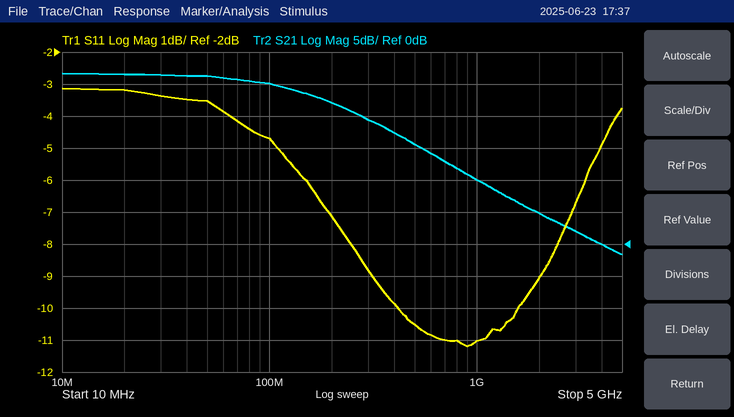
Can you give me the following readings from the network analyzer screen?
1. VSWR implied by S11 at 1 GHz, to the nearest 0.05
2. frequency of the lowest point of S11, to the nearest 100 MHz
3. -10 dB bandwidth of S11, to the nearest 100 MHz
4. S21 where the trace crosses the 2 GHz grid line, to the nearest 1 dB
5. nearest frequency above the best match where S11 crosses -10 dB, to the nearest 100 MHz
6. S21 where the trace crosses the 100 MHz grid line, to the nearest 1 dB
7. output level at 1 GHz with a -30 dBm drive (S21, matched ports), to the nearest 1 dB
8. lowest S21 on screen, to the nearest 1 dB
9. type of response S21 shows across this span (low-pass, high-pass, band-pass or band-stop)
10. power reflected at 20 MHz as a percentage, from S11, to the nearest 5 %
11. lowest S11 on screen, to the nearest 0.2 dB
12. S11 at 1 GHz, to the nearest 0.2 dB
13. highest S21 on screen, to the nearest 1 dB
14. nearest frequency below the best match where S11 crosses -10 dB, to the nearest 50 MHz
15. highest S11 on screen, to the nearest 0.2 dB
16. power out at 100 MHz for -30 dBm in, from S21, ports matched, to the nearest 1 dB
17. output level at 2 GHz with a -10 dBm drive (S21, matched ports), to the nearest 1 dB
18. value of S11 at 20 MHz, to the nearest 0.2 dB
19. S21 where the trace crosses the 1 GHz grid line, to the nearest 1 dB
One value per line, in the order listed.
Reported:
1.80
900 MHz
1.2 GHz
5 dB
1.6 GHz
25 dB
-20 dBm
-2 dB
low-pass
50 %
-11.2 dB
-11.0 dB
27 dB
400 MHz
-3.2 dB
-5 dBm
-5 dBm
-3.2 dB
10 dB
